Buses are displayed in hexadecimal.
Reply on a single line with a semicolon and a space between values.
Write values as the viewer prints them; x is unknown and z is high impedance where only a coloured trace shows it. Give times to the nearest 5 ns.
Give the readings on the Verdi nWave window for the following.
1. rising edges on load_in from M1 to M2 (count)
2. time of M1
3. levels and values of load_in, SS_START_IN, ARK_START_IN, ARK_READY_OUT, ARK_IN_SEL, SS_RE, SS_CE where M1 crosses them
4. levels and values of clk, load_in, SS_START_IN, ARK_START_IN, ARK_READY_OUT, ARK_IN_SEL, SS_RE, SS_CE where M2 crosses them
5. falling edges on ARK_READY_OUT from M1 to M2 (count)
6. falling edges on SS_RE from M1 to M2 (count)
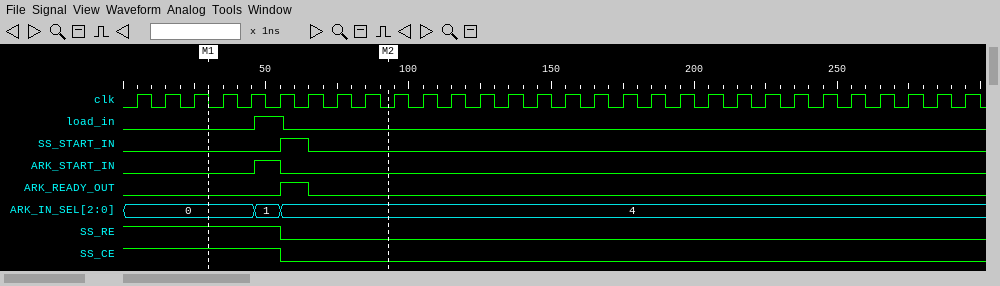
1; 30 ns; load_in=0, SS_START_IN=0, ARK_START_IN=0, ARK_READY_OUT=0, ARK_IN_SEL=0, SS_RE=1, SS_CE=1; clk=0, load_in=0, SS_START_IN=0, ARK_START_IN=0, ARK_READY_OUT=0, ARK_IN_SEL=4, SS_RE=0, SS_CE=0; 1; 1
